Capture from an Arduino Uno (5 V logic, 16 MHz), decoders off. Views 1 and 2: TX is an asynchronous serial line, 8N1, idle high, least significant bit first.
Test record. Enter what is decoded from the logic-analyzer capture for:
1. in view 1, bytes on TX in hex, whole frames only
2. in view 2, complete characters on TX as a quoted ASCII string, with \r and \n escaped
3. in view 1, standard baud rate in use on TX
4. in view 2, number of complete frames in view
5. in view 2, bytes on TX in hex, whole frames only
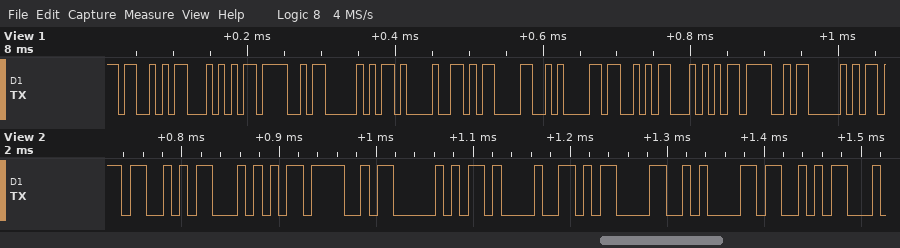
0x53 0x54 0x4F 0x50 0x21 0x0D 0x0A 0x53 0x54 0x4F 0x50
"STOP!\r\nS"
115200 baud
8
53 54 4F 50 21 0D 0A 53
